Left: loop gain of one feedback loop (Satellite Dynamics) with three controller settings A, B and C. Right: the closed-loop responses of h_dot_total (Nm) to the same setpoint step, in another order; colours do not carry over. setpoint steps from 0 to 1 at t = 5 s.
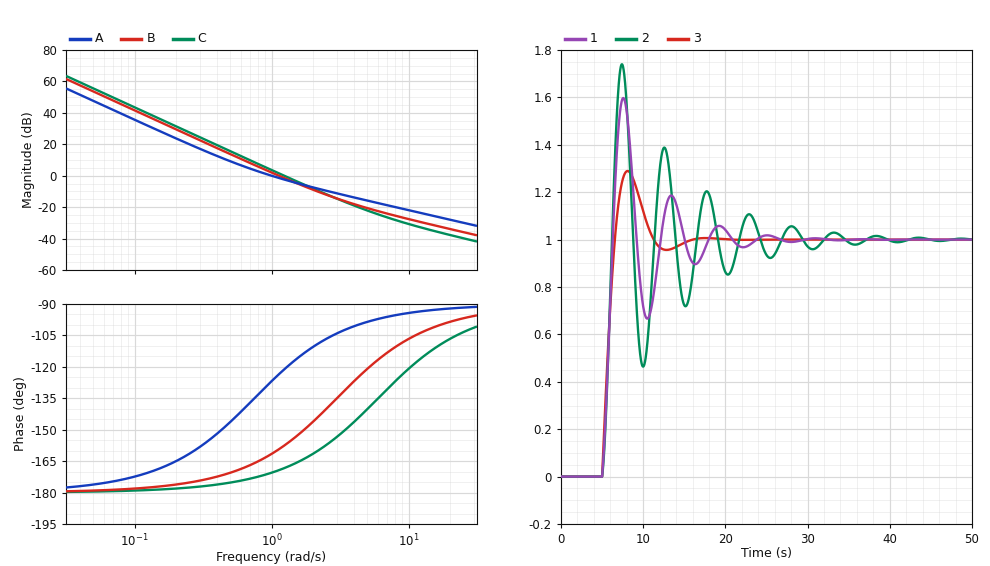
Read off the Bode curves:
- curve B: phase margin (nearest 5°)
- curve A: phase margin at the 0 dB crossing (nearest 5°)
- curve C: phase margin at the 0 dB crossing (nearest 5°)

20°
55°
10°
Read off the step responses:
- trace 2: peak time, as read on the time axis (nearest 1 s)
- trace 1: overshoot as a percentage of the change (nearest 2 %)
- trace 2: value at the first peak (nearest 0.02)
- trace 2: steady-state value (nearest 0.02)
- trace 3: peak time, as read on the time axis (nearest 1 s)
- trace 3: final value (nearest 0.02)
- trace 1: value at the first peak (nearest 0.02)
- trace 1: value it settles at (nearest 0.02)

7 s
60 %
1.74
1.00
8 s
1.00
1.60
1.00
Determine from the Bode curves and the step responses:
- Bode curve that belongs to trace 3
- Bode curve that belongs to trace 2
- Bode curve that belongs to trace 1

A
C
B
